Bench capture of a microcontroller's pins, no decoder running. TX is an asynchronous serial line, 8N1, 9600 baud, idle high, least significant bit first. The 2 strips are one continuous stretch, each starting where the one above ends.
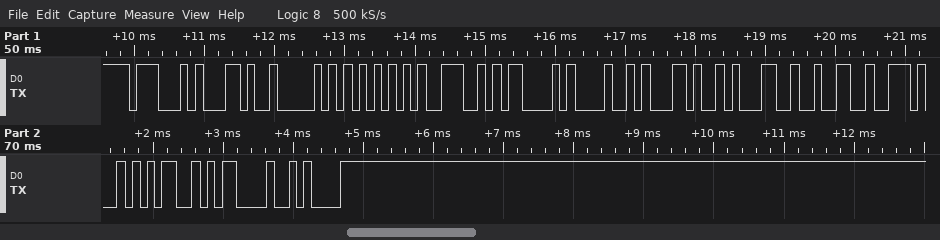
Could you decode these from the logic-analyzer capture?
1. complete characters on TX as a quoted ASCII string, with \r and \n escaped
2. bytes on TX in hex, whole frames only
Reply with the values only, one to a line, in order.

"G,PUNCH,12.5\r\n"
0x47 0x2C 0x50 0x55 0x4E 0x43 0x48 0x2C 0x31 0x32 0x2E 0x35 0x0D 0x0A
